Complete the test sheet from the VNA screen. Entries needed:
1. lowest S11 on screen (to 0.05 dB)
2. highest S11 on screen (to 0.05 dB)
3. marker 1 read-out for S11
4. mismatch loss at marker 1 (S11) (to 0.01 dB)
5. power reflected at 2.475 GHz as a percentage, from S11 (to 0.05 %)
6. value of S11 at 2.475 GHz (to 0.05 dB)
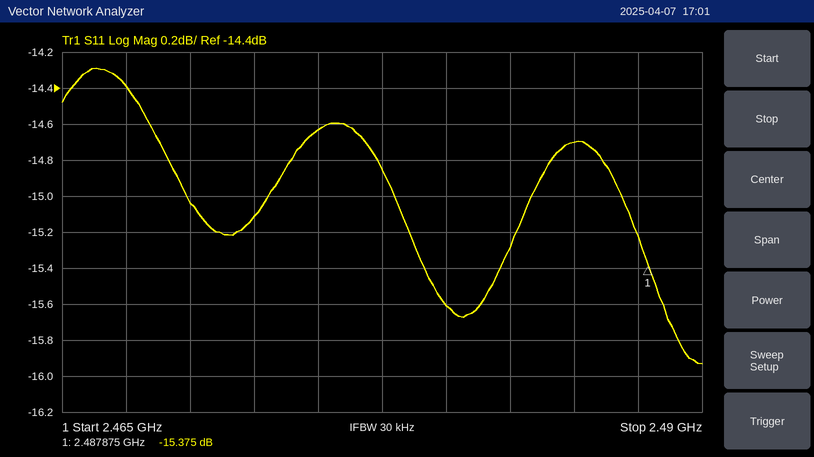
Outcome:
-15.95 dB
-14.30 dB
-15.375 dB
0.13 dB
3.45 %
-14.65 dB
